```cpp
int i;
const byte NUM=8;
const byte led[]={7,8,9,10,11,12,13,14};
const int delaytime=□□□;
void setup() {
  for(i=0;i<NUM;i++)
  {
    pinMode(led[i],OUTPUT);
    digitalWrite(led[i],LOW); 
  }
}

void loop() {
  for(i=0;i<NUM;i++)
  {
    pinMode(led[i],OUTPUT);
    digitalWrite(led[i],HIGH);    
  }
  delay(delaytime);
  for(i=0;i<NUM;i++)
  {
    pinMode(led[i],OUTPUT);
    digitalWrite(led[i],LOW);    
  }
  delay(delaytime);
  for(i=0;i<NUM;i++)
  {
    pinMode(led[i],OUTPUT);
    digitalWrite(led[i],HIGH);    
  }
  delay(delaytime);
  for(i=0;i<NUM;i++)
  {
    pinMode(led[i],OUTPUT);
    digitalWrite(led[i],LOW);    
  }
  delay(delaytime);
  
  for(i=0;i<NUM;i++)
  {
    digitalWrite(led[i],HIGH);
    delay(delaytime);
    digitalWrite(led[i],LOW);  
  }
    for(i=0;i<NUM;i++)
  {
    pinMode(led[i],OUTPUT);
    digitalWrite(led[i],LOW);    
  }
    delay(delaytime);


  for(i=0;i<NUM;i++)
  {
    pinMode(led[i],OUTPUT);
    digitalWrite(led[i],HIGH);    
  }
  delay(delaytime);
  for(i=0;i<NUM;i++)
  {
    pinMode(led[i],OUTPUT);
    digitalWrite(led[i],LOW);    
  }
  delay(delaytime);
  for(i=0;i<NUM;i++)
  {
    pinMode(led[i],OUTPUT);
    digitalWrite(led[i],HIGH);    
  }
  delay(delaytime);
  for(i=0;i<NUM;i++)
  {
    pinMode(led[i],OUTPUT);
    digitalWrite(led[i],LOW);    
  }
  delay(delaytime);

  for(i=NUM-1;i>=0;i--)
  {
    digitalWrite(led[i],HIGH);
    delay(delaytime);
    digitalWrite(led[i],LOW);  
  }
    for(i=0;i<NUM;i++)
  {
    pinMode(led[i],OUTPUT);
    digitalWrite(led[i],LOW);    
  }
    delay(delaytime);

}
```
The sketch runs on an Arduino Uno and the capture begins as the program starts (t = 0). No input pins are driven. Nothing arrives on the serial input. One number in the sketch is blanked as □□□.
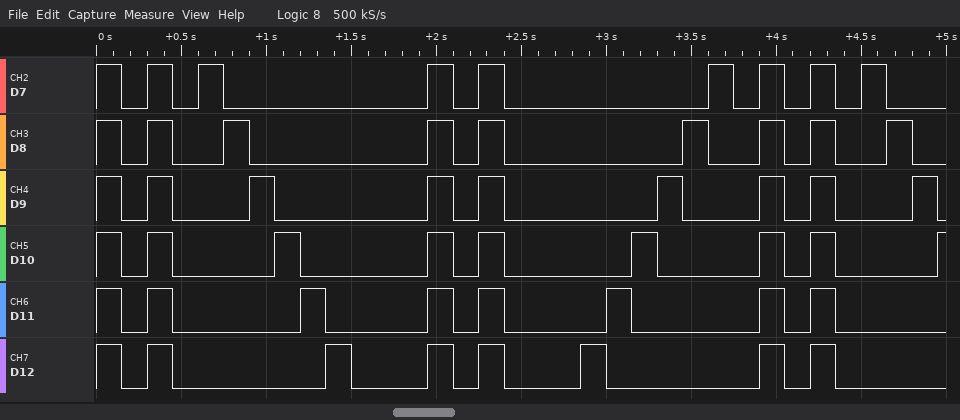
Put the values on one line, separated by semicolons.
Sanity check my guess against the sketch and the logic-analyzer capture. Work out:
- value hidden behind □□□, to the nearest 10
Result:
150
